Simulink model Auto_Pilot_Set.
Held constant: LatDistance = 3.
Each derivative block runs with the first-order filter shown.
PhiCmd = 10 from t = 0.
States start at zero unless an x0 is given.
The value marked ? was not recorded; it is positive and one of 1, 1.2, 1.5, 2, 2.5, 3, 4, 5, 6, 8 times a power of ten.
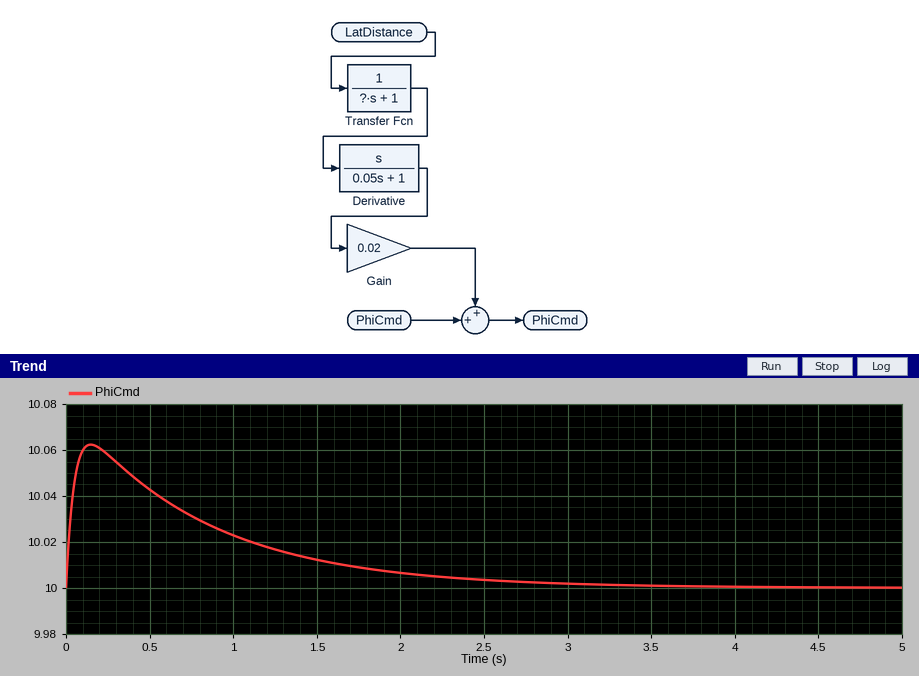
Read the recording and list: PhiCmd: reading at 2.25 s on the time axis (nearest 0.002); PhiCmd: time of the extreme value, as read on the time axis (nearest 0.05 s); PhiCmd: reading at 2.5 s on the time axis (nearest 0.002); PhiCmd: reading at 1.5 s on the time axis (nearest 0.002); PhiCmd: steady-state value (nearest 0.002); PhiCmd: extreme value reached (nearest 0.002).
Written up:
10.004
0.15 s
10.004
10.012
10.000
10.062
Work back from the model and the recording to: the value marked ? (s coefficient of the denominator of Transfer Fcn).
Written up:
0.8
